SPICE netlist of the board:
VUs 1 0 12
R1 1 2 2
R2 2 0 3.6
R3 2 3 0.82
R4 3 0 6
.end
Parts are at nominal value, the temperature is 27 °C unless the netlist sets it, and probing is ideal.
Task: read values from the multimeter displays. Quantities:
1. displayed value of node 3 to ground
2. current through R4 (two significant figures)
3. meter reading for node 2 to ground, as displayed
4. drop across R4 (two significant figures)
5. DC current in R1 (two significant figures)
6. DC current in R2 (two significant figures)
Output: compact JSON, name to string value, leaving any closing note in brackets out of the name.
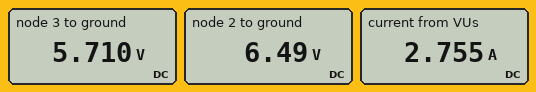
{"displayed value of node 3 to ground": "5.710 V", "current through R4": "950 mA", "meter reading for node 2 to ground, as displayed": "6.49 V", "drop across R4": "5.7 V", "DC current in R1": "2.8 A", "DC current in R2": "1.8 A"}
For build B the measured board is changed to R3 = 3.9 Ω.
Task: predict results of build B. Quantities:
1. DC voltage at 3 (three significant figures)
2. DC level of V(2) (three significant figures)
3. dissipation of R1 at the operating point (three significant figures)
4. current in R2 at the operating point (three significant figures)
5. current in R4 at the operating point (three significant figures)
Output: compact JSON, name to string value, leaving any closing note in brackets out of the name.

{"DC voltage at 3": "4.14 V", "DC level of V(2)": "6.83 V", "dissipation of R1 at the operating point": "13.4 W", "current in R2 at the operating point": "1.90 A", "current in R4 at the operating point": "690 mA"}
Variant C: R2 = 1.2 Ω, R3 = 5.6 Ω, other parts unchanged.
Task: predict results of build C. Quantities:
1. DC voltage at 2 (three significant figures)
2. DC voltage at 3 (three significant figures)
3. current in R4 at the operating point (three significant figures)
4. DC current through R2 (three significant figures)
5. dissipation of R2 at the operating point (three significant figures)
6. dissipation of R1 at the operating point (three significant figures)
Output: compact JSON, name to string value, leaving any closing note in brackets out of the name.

{"DC voltage at 2": "4.23 V", "DC voltage at 3": "2.19 V", "current in R4 at the operating point": "364 mA", "DC current through R2": "3.52 A", "dissipation of R2 at the operating point": "14.9 W", "dissipation of R1 at the operating point": "30.2 W"}
